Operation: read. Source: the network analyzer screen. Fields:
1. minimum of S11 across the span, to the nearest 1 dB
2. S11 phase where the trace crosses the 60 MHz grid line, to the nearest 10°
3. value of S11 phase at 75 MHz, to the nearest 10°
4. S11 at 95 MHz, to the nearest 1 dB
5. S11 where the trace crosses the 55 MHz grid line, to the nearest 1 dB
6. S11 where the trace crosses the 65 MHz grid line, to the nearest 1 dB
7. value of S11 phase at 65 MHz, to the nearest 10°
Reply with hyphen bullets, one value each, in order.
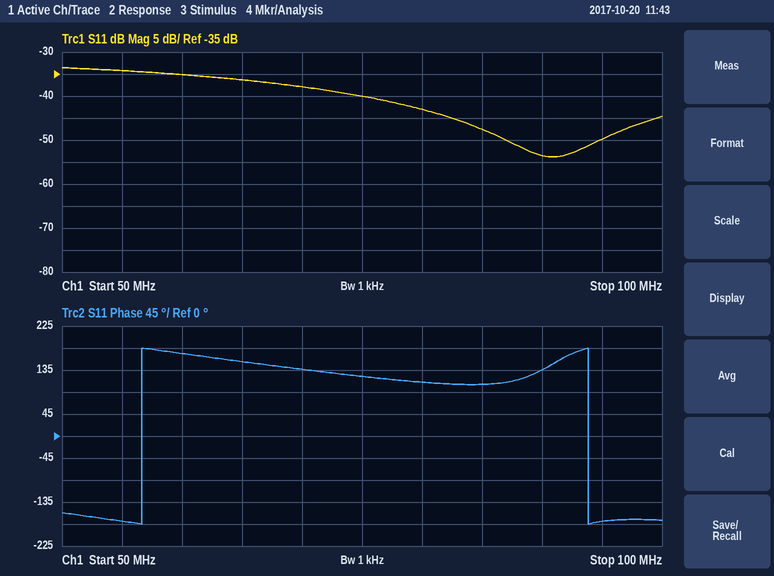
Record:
- -54 dB
- 170°
- 120°
- -50 dB
- -34 dB
- -36 dB
- 150°
